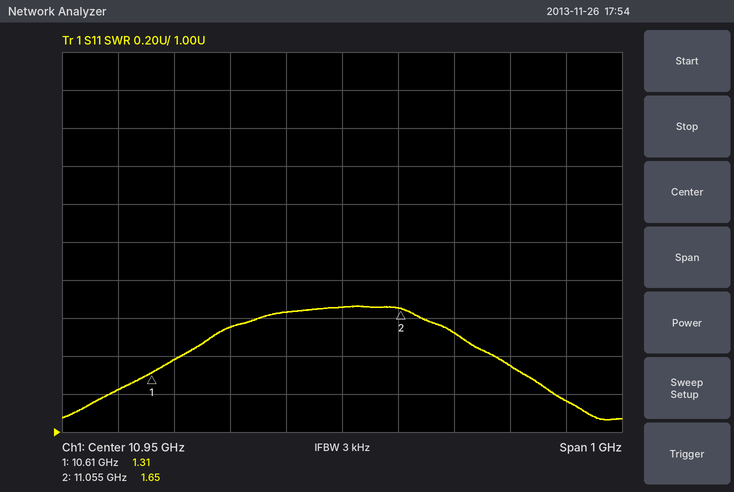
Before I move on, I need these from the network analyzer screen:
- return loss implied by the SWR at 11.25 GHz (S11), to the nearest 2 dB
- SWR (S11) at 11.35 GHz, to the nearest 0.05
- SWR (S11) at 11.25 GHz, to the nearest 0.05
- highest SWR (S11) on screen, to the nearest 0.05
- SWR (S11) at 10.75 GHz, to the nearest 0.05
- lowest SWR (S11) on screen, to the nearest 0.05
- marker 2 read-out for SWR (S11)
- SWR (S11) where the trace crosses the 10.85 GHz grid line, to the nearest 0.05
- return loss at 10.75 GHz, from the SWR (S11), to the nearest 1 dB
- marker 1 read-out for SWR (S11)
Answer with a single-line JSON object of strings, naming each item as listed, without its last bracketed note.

{"return loss implied by the SWR at 11.25 GHz (S11), to the nearest 2 dB": "16 dB", "SWR (S11) at 11.35 GHz, to the nearest 0.05": "1.15", "SWR (S11) at 11.25 GHz, to the nearest 0.05": "1.35", "highest SWR (S11) on screen, to the nearest 0.05": "1.65", "SWR (S11) at 10.75 GHz, to the nearest 0.05": "1.55", "lowest SWR (S11) on screen, to the nearest 0.05": "1.05", "marker 2 read-out for SWR": "1.65", "SWR (S11) where the trace crosses the 10.85 GHz grid line, to the nearest 0.05": "1.65", "return loss at 10.75 GHz, from the SWR (S11), to the nearest 1 dB": "13 dB", "marker 1 read-out for SWR": "1.31"}
